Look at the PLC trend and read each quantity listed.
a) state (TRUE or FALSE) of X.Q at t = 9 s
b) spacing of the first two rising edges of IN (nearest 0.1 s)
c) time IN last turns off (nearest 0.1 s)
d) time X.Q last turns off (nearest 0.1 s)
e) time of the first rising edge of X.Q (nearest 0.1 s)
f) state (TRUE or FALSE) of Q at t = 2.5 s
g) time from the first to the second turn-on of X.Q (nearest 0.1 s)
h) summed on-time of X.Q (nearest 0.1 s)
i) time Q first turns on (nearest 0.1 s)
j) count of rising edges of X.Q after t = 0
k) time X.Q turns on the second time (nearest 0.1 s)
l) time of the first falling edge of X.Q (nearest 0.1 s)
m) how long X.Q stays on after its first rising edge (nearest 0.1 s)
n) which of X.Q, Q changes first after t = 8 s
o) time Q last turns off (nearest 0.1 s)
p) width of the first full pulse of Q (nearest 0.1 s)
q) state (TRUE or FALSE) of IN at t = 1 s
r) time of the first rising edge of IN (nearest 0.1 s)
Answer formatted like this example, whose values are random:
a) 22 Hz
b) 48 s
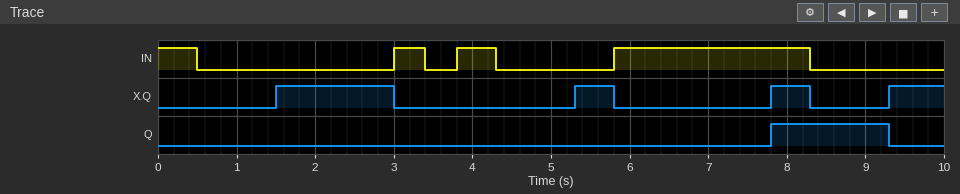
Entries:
a) FALSE
b) 0.8 s
c) 8.3 s
d) 8.3 s
e) 1.5 s
f) FALSE
g) 3.8 s
h) 3.2 s
i) 7.8 s
j) 4
k) 5.3 s
l) 3.0 s
m) 1.5 s
n) X.Q
o) 9.3 s
p) 1.5 s
q) FALSE
r) 3.0 s
